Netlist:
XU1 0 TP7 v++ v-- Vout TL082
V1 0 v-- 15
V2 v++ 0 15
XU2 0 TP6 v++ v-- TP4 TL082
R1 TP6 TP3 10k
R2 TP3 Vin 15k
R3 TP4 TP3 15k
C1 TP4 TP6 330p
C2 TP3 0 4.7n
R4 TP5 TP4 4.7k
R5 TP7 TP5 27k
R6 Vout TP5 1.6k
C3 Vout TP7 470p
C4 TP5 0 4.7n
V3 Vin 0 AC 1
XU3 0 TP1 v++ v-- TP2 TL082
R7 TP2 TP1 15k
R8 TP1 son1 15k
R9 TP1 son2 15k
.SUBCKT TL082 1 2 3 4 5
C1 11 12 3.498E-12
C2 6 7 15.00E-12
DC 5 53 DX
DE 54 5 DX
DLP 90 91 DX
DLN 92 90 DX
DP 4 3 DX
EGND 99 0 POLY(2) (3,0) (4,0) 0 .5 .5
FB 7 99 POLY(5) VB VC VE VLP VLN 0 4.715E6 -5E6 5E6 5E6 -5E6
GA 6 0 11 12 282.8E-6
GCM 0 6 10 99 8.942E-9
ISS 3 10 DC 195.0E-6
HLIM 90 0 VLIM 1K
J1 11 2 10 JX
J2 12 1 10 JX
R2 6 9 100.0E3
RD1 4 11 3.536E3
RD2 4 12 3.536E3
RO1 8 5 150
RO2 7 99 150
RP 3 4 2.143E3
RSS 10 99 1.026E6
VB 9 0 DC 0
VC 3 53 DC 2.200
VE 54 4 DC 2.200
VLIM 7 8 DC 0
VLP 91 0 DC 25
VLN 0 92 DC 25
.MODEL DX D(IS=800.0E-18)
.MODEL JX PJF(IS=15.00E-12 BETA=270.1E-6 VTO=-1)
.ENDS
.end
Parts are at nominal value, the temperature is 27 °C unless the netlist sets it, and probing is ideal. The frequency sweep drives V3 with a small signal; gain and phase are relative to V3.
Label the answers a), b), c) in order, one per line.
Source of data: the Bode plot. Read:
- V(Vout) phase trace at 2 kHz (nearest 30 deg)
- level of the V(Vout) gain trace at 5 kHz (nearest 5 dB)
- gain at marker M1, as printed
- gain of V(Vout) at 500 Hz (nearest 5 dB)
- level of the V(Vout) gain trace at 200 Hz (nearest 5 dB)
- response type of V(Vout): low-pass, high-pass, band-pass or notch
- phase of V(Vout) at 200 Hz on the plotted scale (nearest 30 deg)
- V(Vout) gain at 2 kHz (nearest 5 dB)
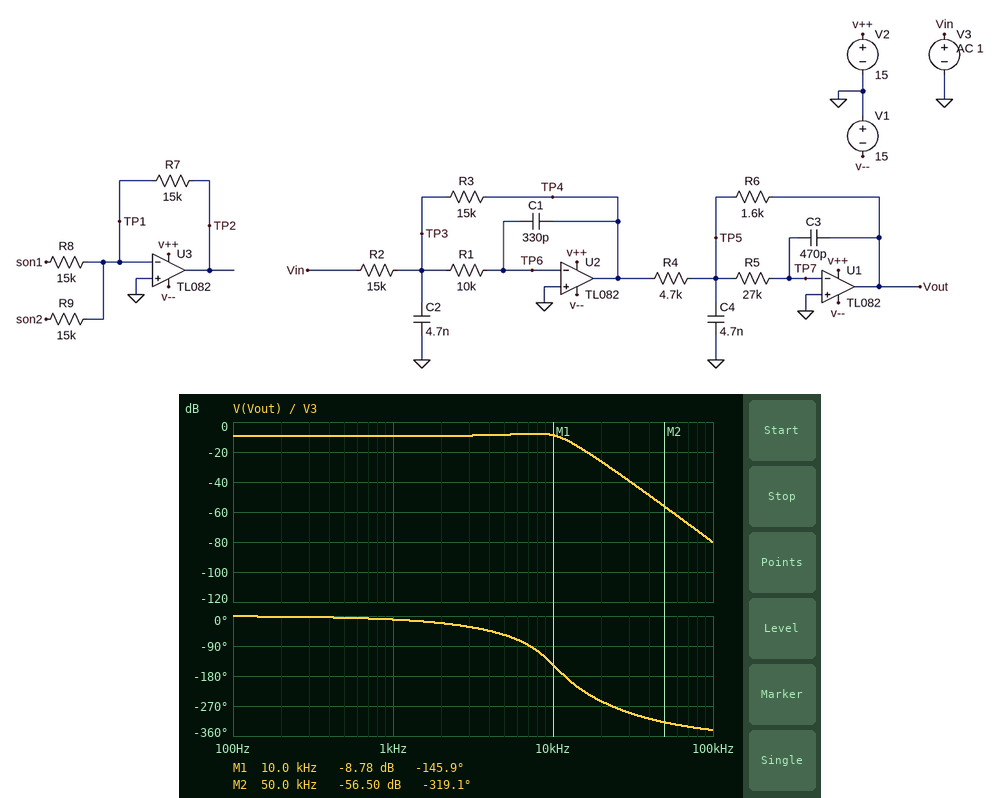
a) -30 deg
b) -10 dB
c) -8.78 dB
d) -10 dB
e) -10 dB
f) low-pass
g) 0 deg
h) -10 dB
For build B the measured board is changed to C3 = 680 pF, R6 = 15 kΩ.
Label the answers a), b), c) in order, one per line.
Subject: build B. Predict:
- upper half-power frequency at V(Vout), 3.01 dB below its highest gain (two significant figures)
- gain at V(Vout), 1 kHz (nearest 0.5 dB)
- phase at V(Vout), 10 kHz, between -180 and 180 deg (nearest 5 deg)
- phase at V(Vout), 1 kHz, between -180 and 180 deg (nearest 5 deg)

a) 2.3 kHz
b) 9.5 dB
c) 150 deg
d) -35 deg
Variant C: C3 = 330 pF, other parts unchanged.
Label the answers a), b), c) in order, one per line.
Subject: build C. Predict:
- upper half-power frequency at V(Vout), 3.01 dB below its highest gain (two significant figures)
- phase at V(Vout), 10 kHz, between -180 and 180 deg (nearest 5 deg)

a) 12 kHz
b) -130 deg
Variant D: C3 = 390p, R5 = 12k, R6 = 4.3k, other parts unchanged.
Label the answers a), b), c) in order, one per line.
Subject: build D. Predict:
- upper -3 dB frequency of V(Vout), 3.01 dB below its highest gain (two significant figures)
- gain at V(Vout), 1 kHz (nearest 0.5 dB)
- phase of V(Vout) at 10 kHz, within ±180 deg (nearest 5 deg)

a) 12 kHz
b) -0.5 dB
c) -130 deg
